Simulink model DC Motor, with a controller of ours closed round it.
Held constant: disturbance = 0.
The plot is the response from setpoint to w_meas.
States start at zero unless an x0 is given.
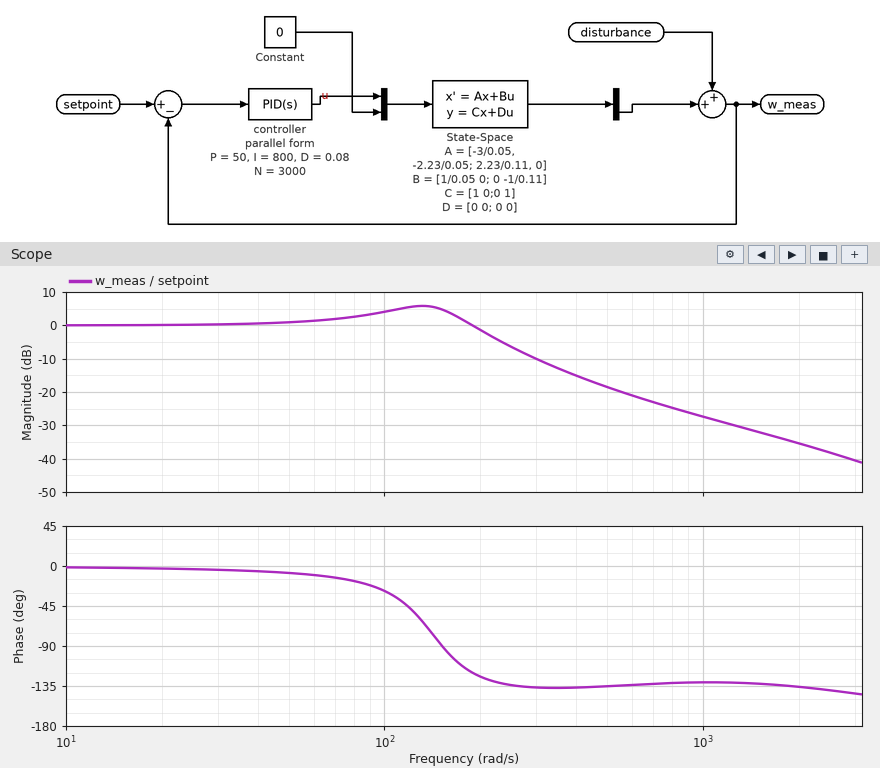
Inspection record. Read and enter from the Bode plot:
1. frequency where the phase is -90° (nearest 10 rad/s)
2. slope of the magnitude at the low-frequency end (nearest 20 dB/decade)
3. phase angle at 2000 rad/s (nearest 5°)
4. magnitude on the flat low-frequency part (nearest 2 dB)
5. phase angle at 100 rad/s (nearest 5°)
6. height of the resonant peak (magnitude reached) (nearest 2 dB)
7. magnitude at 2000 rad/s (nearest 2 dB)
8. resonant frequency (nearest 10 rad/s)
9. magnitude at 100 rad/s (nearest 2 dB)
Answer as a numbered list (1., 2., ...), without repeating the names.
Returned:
1. 150 rad/s
2. 0 dB/decade
3. -135°
4. 0 dB
5. -30°
6. 6 dB
7. -36 dB
8. 130 rad/s
9. 4 dB
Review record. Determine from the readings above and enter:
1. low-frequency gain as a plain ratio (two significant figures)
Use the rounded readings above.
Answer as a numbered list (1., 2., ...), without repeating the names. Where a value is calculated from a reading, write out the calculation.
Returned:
1. 10^(0 / 20) = 1.0
